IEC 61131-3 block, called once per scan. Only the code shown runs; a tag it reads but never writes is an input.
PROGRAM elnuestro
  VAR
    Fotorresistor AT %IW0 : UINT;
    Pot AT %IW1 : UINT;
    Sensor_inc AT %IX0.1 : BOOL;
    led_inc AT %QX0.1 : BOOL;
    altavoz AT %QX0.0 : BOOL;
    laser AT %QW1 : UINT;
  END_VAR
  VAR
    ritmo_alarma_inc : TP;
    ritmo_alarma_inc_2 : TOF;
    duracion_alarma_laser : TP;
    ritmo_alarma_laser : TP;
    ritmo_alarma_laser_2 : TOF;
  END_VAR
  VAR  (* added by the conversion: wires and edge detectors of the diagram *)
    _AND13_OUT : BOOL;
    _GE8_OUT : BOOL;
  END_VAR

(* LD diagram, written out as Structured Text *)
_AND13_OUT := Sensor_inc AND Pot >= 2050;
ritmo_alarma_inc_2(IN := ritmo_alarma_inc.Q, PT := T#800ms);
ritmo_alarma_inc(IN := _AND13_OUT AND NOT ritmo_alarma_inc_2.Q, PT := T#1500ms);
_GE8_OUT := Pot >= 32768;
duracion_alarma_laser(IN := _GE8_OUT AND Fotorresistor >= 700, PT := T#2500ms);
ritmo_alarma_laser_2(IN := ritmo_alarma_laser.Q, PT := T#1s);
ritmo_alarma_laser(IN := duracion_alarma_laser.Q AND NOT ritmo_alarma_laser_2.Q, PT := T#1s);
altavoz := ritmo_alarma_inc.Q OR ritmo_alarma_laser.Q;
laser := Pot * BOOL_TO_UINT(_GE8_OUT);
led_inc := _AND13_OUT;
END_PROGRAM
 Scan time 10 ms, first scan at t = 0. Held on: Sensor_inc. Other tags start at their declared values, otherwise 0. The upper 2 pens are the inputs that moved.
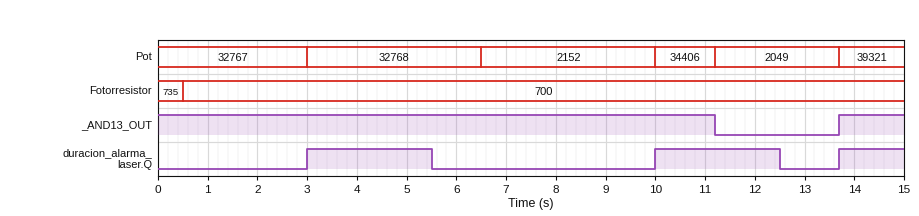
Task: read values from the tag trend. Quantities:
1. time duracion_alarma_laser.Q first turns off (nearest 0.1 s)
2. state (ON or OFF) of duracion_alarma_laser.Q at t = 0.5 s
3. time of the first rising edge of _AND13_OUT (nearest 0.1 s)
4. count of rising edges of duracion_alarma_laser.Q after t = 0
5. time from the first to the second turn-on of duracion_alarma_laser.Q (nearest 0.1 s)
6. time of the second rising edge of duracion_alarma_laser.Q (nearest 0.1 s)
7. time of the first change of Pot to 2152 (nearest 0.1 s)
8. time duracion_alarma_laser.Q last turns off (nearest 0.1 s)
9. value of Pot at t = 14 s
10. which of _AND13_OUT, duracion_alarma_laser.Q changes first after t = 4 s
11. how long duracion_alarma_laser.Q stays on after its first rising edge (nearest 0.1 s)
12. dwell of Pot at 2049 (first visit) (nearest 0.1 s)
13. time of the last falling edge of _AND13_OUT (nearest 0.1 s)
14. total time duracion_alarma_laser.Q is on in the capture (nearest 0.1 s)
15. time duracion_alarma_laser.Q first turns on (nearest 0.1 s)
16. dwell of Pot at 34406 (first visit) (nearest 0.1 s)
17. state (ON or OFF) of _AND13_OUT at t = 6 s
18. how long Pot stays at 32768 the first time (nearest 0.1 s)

5.5 s
OFF
13.7 s
3
7.0 s
10.0 s
6.5 s
12.5 s
39321
duracion_alarma_laser.Q
2.5 s
2.5 s
11.2 s
6.3 s
3.0 s
1.2 s
ON
3.5 s
